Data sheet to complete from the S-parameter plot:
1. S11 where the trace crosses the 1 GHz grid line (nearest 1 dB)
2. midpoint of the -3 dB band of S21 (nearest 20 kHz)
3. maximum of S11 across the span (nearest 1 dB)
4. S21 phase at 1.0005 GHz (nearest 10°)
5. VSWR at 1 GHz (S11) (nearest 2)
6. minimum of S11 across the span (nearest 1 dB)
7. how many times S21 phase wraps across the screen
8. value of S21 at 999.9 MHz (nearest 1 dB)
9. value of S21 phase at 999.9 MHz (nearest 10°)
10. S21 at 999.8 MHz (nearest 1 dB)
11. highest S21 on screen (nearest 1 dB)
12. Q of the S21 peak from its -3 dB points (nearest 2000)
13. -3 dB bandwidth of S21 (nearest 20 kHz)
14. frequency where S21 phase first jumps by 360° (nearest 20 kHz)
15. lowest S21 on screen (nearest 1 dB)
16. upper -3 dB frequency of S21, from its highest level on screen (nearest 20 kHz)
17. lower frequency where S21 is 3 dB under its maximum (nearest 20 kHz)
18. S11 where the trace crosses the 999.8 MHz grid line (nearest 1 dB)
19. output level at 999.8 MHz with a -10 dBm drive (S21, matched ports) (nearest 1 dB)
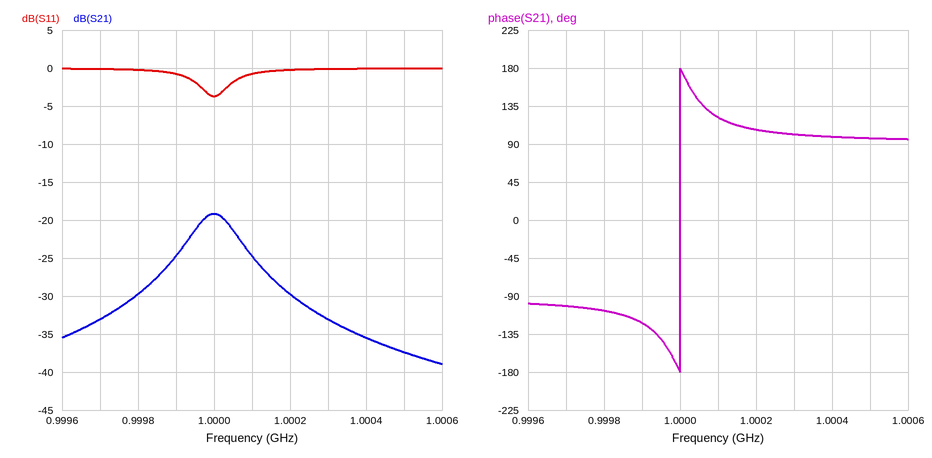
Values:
-4 dB
1.00000 GHz
0 dB
100°
4
-4 dB
1
-25 dB
-120°
-30 dB
-19 dB
8000
120 kHz
1.00000 GHz
-39 dB
1.00006 GHz
999.94 MHz
0 dB
-40 dBm
